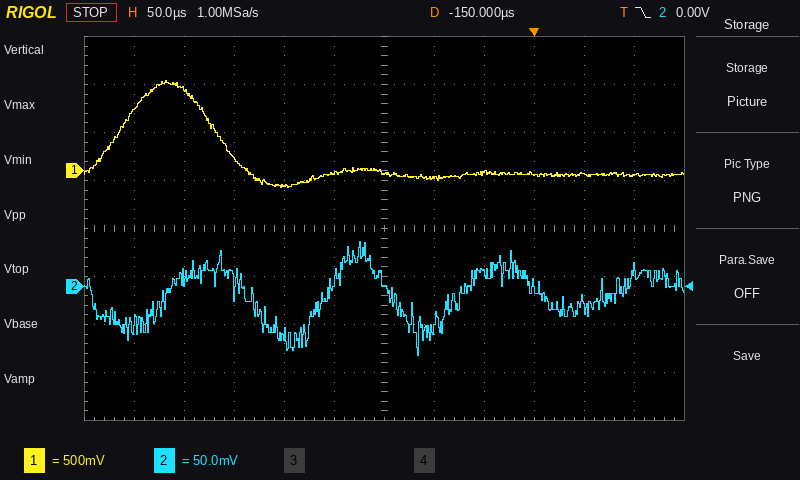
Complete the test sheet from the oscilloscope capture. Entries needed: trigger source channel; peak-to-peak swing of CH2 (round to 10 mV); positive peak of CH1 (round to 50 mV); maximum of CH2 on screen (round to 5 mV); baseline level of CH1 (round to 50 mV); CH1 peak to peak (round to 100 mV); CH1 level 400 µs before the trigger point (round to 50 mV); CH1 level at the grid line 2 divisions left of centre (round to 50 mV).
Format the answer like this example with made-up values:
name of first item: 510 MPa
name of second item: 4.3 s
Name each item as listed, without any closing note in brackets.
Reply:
trigger source channel: CH2
peak-to-peak swing of CH2: 120 mV
positive peak of CH1: 950 mV
maximum of CH2 on screen: 45 mV
baseline level of CH1: -50 mV
CH1 peak to peak: 1.10 V
CH1 level 400 µs before the trigger point: 650 mV
CH1 level at the grid line 2 divisions left of centre: -150 mV
